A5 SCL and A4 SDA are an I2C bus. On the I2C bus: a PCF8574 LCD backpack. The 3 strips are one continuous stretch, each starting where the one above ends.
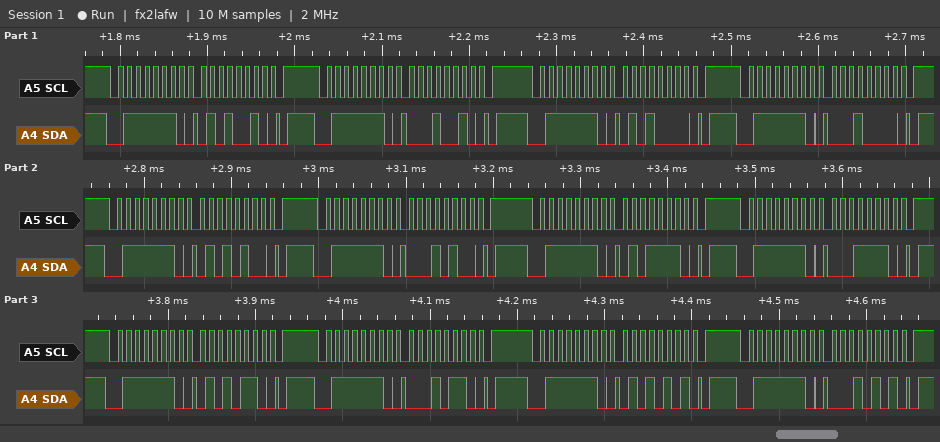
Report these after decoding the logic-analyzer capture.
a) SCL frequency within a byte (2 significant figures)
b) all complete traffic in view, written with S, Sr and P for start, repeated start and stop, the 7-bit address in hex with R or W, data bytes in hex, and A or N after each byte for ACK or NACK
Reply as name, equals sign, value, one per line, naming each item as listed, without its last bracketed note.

SCL frequency within a byte = 100 kHz
all complete traffic in view, written with S, Sr and P for start, repeated start and stop, the 7-bit address in hex with R or W, data bytes in hex, and A or N after each byte for ACK or NACK = S 3FW A 52 A P S 3FW A 12 A P S 3FW A 50 A P S 3FW A 10 A P S 3FW A 54 A P S 3FW A 14 A P S 3FW A 5E A P S 3FW A 1E A P S 3FW A 56 A P S 3FW A 16 A P S 3FW A 55 A P S 3FW A 15 A P
